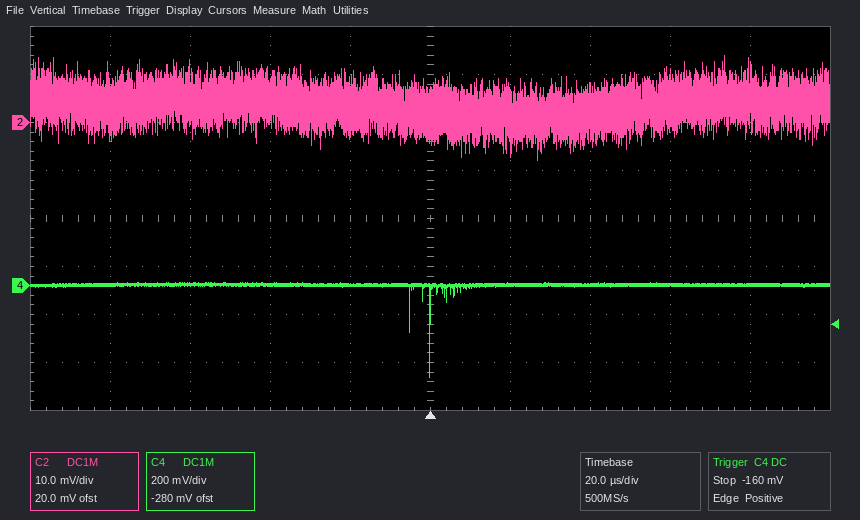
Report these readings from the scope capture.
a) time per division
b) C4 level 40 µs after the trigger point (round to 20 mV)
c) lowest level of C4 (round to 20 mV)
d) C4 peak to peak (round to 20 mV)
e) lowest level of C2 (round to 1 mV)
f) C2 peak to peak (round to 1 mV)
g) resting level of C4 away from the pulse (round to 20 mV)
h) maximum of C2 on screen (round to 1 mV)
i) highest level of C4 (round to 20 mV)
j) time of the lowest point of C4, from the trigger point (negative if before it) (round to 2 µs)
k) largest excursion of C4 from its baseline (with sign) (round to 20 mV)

20 µs
0 mV
-380 mV
400 mV
-8 mV
22 mV
0 mV
14 mV
20 mV
0 µs
-380 mV
